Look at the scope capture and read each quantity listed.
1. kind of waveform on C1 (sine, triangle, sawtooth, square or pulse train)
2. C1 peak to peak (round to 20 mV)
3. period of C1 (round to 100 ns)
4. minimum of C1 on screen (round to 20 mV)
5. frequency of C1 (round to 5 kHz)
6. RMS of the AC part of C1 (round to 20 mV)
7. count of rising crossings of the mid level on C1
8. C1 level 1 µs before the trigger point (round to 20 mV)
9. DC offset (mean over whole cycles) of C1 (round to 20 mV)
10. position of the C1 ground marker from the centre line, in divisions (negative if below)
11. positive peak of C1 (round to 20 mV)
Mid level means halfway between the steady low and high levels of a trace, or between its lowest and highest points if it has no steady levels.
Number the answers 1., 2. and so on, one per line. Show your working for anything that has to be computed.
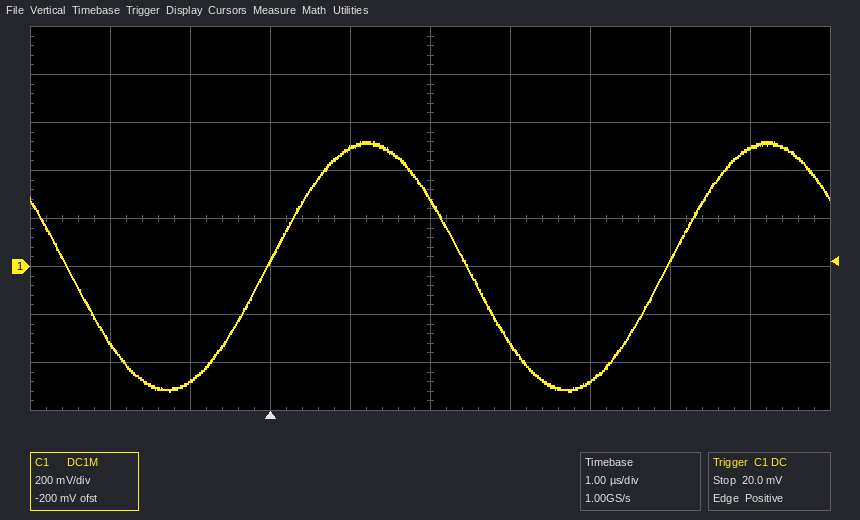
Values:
1. sine
2. 520 mV − (-520 mV) = 1.04 V
3. 5.0 µs
4. -520 mV
5. 1 / 5.0 µs ≈ 200 kHz
6. 1.04 V / (2√2) ≈ 368 mV, so 360 mV to the nearest 20 mV
7. 2
8. -480 mV
9. (520 mV + (-520 mV)) / 2 ≈ 0 mV
10. -1.0 div
11. 520 mV
